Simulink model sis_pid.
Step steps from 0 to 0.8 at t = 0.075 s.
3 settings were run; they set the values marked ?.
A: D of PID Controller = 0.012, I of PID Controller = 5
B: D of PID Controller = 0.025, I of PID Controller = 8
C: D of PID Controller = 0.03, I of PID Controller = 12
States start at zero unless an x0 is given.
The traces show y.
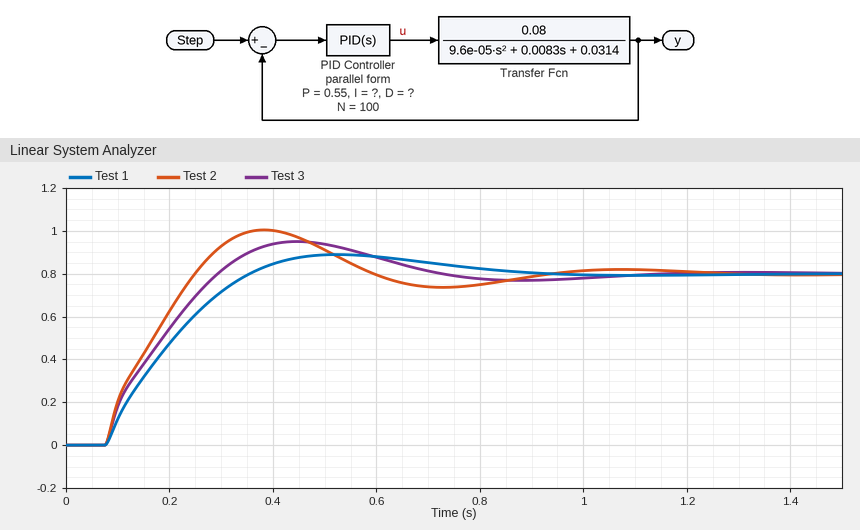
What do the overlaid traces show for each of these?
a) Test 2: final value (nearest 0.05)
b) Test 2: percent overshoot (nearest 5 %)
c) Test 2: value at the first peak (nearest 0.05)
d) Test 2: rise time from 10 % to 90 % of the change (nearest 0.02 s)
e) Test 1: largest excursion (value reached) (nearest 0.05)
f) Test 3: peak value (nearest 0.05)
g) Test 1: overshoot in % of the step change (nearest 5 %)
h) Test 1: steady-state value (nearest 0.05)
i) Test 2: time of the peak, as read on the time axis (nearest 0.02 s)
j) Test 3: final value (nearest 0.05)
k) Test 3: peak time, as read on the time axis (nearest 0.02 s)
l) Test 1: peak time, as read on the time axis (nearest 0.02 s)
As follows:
0.80
25 %
1.00
0.14 s
0.90
0.95
10 %
0.80
0.38 s
0.80
0.44 s
0.52 s
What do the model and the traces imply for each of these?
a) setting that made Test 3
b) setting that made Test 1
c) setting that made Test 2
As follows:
B
A
C
